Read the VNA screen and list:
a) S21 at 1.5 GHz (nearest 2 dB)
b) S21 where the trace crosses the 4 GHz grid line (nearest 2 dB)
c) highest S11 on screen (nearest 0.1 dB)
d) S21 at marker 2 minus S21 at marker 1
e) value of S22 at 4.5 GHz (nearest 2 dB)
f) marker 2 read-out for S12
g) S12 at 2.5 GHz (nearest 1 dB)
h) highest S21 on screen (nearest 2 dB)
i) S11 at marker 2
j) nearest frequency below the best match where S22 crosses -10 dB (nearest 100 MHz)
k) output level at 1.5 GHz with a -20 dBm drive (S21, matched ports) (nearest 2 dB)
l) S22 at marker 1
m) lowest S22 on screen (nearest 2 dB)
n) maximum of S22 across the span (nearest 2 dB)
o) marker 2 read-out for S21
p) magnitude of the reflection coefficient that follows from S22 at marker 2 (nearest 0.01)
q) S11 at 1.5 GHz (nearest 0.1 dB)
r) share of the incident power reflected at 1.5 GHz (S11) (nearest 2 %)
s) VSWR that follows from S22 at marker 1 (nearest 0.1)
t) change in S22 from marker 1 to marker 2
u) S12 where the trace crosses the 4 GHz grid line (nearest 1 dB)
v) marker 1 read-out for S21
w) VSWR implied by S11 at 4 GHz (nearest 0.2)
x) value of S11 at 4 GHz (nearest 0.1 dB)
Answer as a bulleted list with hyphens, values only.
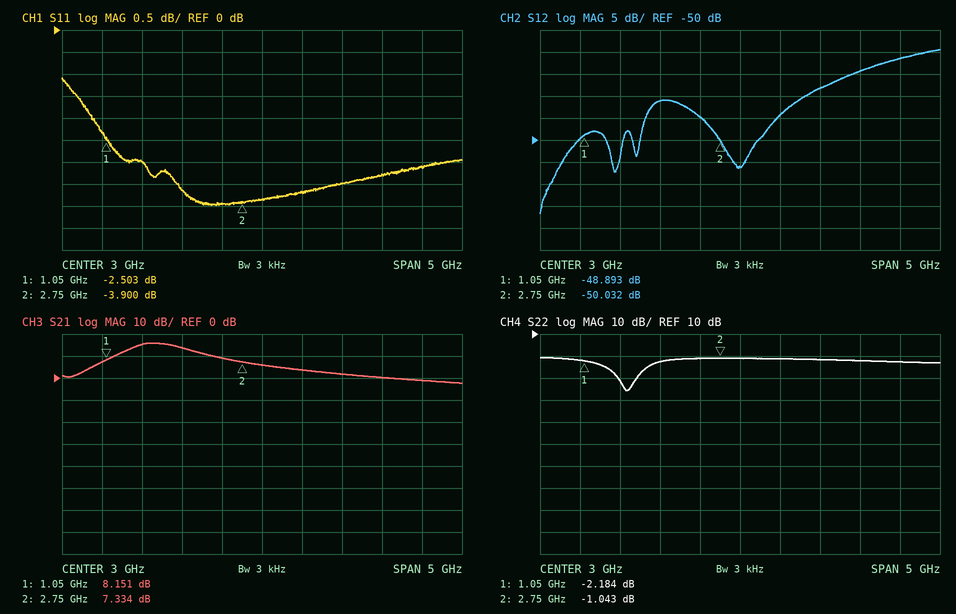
- 16 dB
- 2 dB
- -1.1 dB
- -0.817 dB
- -2 dB
- -50.032 dB
- -45 dB
- 16 dB
- -3.900 dB
- 1.5 GHz
- -4 dBm
- -2.184 dB
- -16 dB
- 0 dB
- 7.334 dB
- 0.89
- -3.0 dB
- 50 %
- 8.0
- 1.141 dB
- -38 dB
- 8.151 dB
- 5.0
- -3.5 dB
